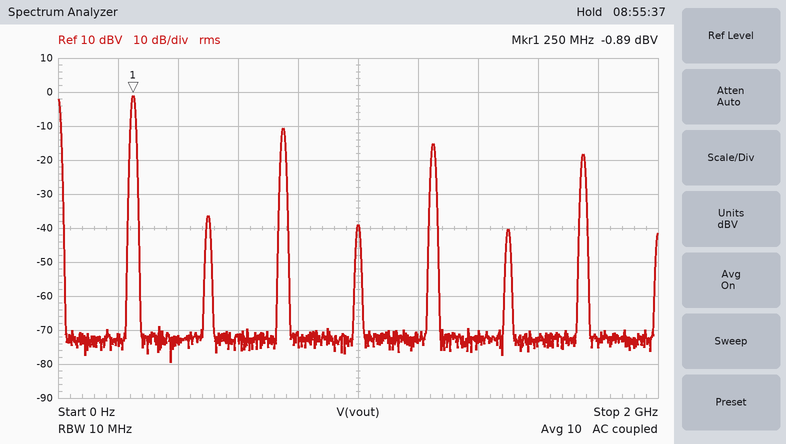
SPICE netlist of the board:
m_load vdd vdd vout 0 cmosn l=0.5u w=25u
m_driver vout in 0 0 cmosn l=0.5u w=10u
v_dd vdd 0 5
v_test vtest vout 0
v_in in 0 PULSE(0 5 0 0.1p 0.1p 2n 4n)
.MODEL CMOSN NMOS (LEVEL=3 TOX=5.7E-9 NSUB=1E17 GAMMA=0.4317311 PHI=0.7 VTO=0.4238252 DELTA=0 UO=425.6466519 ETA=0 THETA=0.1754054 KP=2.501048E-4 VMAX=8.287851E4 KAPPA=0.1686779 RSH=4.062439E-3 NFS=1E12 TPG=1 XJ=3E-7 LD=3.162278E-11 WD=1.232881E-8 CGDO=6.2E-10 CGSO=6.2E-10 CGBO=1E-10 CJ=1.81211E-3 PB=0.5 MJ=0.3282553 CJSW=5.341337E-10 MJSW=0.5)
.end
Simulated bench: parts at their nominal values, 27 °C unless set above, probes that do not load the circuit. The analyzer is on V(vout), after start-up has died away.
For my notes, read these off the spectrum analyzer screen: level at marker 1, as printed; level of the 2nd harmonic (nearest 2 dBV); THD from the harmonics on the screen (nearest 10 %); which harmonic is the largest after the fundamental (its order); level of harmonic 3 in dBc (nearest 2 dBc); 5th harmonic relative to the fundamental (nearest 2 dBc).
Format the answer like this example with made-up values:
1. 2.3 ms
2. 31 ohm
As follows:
1. -0.89 dBV
2. -36 dBV
3. 40 %
4. 3
5. -10 dBc
6. -14 dBc
